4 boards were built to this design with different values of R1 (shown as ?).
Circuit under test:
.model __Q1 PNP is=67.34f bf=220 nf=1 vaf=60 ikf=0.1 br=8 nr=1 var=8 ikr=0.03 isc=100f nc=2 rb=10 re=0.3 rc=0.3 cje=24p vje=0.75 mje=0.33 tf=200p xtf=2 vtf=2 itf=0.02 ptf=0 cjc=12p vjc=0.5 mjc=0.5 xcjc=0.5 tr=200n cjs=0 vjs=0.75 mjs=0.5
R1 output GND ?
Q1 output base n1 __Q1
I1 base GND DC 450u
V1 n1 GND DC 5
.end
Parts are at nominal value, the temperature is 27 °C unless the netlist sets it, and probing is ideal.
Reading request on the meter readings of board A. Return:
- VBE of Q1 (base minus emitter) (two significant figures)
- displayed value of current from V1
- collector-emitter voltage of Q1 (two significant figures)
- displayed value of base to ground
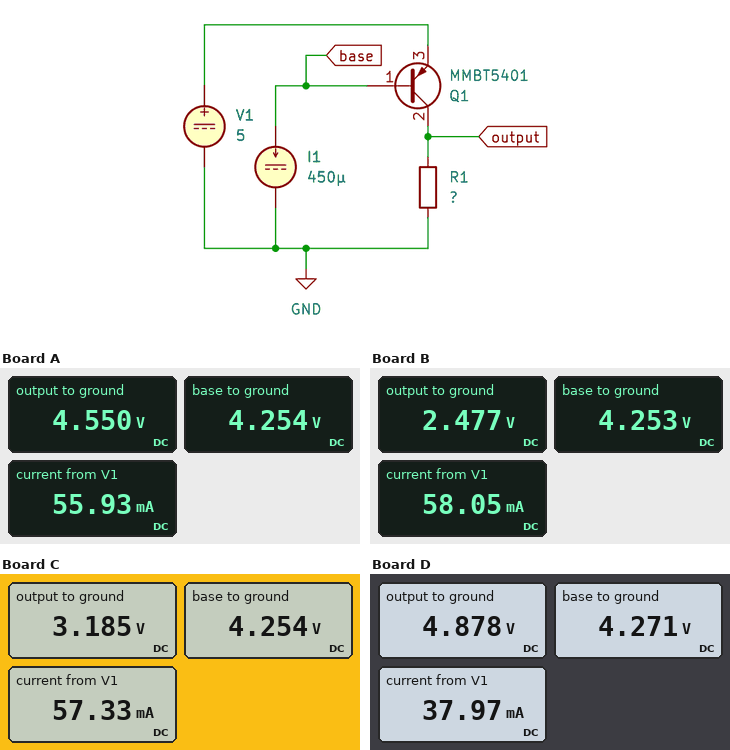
-750 mV
55.93 mA
-450 mV
4.254 V
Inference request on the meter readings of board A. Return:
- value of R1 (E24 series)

82 Ω
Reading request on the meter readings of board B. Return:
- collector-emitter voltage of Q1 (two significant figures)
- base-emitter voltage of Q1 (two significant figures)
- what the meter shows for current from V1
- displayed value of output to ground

-2.5 V
-750 mV
58.05 mA
2.477 V
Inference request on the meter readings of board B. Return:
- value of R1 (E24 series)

43 Ω
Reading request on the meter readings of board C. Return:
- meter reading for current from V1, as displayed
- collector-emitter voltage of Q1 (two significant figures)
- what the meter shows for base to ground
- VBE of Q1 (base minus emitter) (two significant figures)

57.33 mA
-1.8 V
4.254 V
-750 mV
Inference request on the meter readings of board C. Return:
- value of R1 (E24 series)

56 Ω
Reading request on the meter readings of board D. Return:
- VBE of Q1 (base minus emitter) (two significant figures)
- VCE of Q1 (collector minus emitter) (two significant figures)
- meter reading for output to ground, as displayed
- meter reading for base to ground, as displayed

-730 mV
-120 mV
4.878 V
4.271 V
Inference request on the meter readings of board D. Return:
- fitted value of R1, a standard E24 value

130 Ω
